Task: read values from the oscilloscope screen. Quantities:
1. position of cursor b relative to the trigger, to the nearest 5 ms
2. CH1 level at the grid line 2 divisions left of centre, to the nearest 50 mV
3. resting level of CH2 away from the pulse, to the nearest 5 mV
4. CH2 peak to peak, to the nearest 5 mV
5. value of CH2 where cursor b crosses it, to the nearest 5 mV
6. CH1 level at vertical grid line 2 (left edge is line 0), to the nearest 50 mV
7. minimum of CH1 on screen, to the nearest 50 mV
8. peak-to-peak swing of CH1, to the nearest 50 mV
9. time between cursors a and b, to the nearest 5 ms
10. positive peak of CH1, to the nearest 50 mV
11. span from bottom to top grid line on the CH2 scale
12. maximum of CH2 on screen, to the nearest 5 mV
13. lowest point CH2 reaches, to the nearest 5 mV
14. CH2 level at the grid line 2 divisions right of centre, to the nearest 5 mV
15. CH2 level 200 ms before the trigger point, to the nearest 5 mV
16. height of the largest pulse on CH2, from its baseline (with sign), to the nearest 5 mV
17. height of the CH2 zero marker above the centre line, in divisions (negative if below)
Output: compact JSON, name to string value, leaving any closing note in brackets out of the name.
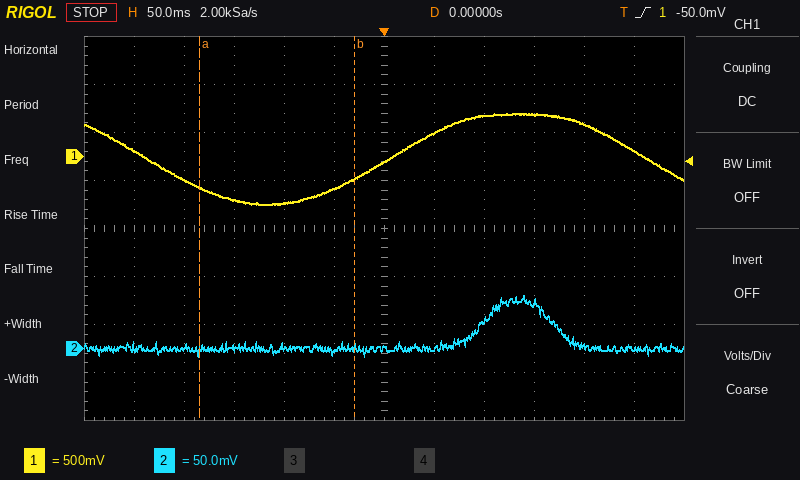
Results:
{"position of cursor b relative to the trigger, to the nearest 5 ms": "-30 ms", "CH1 level at the grid line 2 divisions left of centre, to the nearest 50 mV": "-500 mV", "resting level of CH2 away from the pulse, to the nearest 5 mV": "0 mV", "CH2 peak to peak, to the nearest 5 mV": "65 mV", "value of CH2 where cursor b crosses it, to the nearest 5 mV": "0 mV", "CH1 level at vertical grid line 2 (left edge is line 0), to the nearest 50 mV": "-250 mV", "minimum of CH1 on screen, to the nearest 50 mV": "-500 mV", "peak-to-peak swing of CH1, to the nearest 50 mV": "950 mV", "time between cursors a and b, to the nearest 5 ms": "155 ms", "positive peak of CH1, to the nearest 50 mV": "450 mV", "span from bottom to top grid line on the CH2 scale": "400 mV", "maximum of CH2 on screen, to the nearest 5 mV": "55 mV", "lowest point CH2 reaches, to the nearest 5 mV": "-10 mV", "CH2 level at the grid line 2 divisions right of centre, to the nearest 5 mV": "30 mV", "CH2 level 200 ms before the trigger point, to the nearest 5 mV": "0 mV", "height of the largest pulse on CH2, from its baseline (with sign), to the nearest 5 mV": "+55 mV", "height of the CH2 zero marker above the centre line, in divisions": "-2.5 div"}
